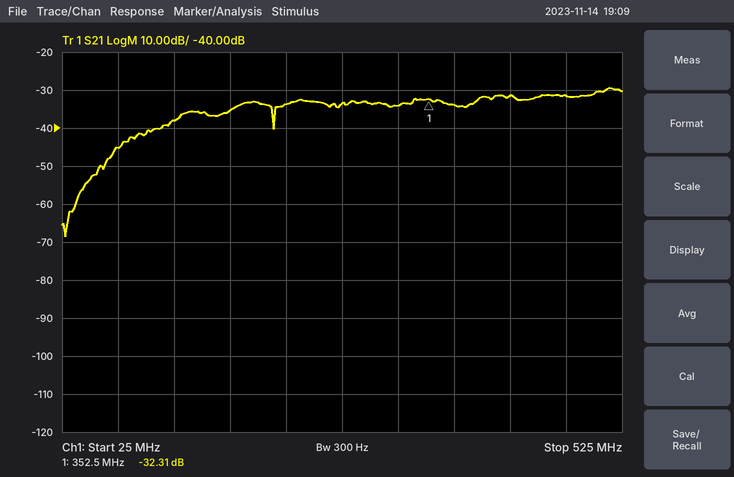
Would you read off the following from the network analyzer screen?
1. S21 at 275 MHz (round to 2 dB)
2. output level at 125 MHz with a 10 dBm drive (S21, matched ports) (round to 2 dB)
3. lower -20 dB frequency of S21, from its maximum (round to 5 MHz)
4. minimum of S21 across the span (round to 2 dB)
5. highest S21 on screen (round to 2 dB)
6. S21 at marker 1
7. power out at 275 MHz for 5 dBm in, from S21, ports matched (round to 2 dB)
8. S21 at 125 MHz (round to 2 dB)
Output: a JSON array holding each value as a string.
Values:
["-34 dB", "-28 dBm", "65 MHz", "-68 dB", "-30 dB", "-32.31 dB", "-28 dBm", "-38 dB"]
